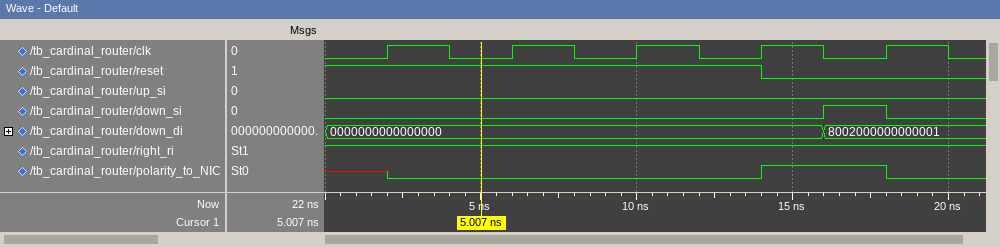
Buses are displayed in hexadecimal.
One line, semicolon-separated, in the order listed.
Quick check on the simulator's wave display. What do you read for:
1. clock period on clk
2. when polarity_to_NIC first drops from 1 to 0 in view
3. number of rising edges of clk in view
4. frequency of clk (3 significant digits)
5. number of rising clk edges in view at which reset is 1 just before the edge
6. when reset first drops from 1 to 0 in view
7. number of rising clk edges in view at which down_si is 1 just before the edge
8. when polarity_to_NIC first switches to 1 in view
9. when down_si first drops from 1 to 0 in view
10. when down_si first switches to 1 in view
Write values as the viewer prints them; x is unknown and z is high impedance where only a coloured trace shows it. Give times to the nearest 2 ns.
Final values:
4 ns; 18 ns; 5; 250 MHz; 4; 14 ns; 1; 14 ns; 18 ns; 16 ns
